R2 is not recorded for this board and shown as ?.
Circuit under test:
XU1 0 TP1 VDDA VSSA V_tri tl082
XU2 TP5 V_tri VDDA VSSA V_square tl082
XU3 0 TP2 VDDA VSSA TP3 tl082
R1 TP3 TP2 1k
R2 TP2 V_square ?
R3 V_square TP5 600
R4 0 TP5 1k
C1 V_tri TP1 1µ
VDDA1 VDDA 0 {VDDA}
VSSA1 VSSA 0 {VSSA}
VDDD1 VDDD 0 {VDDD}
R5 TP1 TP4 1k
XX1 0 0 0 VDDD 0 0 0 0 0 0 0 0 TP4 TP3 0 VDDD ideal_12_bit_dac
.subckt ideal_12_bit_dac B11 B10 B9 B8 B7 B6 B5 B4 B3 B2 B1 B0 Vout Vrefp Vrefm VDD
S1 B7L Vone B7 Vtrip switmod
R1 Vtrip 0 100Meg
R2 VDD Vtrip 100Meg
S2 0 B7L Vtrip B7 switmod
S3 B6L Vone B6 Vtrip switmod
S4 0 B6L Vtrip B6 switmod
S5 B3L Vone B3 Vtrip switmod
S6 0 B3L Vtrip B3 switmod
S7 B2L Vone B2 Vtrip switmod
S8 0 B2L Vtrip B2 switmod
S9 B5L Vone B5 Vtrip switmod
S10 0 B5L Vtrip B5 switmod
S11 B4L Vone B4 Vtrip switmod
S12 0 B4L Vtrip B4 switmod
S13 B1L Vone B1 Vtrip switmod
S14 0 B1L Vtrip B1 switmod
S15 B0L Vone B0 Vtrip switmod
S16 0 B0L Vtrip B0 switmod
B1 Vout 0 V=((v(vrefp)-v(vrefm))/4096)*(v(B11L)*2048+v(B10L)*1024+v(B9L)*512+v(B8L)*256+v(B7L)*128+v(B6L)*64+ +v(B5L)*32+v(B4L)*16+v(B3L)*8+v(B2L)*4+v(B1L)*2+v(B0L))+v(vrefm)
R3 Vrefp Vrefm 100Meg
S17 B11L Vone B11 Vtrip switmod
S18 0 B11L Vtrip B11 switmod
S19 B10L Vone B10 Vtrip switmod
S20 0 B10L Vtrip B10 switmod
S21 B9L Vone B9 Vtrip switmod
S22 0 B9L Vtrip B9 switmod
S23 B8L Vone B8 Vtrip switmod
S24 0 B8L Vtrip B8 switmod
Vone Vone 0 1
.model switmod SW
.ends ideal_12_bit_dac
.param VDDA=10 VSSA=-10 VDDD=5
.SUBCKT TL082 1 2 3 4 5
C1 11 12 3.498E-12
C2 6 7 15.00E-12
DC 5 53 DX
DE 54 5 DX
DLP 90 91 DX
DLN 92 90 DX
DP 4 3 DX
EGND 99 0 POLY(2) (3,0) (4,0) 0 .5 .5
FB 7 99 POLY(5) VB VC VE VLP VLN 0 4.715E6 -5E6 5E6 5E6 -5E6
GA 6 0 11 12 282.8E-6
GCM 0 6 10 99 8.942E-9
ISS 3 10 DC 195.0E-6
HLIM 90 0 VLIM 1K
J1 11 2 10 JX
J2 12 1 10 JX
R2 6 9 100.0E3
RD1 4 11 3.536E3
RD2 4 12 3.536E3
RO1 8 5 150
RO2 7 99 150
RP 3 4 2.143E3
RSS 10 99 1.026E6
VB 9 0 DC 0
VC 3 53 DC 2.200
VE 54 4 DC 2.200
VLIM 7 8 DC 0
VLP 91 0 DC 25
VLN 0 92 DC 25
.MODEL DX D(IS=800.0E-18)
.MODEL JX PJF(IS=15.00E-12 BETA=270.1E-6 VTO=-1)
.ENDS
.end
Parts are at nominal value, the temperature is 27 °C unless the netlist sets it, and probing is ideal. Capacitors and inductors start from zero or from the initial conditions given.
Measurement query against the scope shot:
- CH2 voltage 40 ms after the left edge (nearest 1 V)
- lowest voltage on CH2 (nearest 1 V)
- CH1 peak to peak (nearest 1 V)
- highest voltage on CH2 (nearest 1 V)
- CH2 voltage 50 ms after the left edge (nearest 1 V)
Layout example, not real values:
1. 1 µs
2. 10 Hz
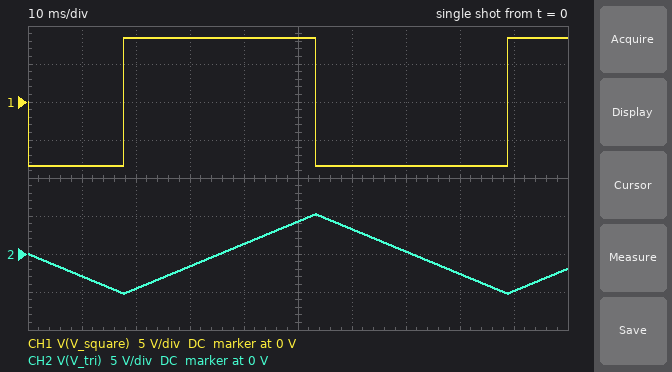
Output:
1. 1 V
2. -5 V
3. 17 V
4. 5 V
5. 4 V
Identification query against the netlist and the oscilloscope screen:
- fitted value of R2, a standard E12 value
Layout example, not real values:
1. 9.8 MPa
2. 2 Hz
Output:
1. 1.8 kΩ
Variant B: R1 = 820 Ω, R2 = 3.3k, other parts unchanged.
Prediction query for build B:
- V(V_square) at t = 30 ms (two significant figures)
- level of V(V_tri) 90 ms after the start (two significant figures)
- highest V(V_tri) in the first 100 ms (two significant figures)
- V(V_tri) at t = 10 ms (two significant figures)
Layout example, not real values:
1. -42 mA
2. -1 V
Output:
1. -8.5 V
2. 1.4 V
3. 2.7 V
4. -1.3 V
